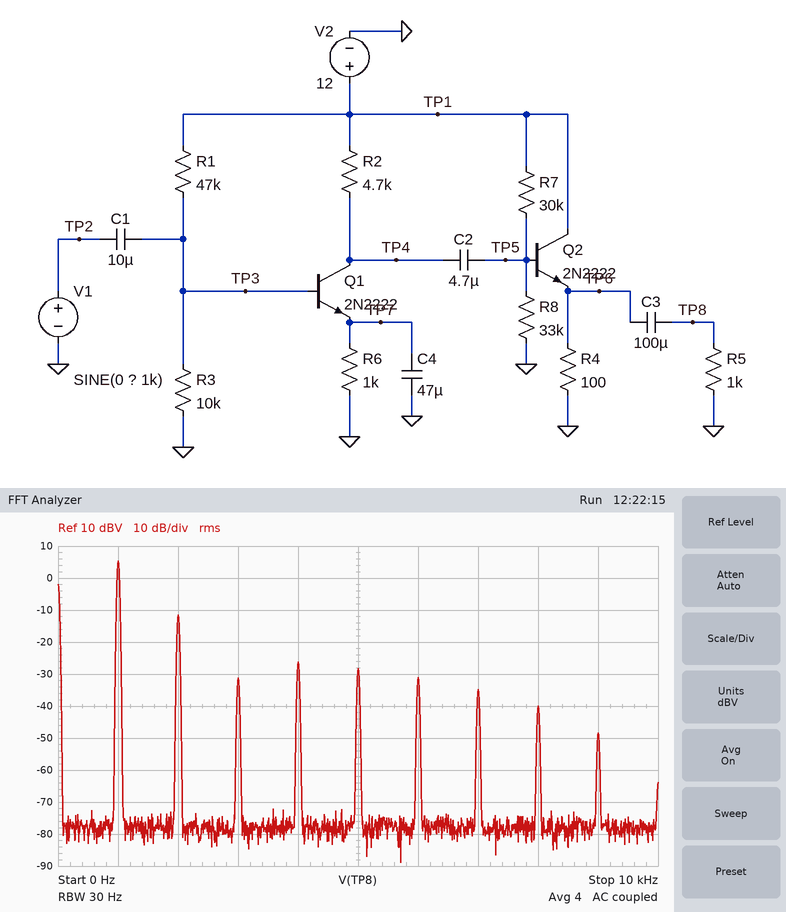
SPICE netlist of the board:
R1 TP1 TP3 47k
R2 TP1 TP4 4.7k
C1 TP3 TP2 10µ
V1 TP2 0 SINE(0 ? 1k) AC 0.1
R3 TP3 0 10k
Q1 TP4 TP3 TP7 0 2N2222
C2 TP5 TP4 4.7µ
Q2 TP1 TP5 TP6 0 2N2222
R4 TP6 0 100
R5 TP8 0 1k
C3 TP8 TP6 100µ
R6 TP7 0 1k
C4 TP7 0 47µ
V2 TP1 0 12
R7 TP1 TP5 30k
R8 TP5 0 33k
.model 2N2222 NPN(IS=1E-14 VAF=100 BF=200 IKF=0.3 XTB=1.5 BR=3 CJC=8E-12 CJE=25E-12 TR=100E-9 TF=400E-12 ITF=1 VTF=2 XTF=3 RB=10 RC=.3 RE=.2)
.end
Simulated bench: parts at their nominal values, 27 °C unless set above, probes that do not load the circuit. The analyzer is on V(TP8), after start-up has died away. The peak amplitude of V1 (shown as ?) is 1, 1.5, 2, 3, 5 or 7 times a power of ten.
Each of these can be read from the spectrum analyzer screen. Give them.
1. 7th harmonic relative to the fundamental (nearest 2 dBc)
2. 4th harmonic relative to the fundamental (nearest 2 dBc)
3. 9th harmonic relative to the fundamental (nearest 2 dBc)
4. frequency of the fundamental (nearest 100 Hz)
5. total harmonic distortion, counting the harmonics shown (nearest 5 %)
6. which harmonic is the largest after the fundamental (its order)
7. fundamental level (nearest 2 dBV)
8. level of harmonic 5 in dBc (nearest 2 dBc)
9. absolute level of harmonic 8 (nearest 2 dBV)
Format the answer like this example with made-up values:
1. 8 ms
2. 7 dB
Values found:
1. -40 dBc
2. -32 dBc
3. -54 dBc
4. 1.0 kHz
5. 15 %
6. 2
7. 6 dBV
8. -34 dBc
9. -40 dBV
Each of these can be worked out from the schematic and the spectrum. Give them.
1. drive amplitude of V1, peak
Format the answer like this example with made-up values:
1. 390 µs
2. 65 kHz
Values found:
1. 20 mV
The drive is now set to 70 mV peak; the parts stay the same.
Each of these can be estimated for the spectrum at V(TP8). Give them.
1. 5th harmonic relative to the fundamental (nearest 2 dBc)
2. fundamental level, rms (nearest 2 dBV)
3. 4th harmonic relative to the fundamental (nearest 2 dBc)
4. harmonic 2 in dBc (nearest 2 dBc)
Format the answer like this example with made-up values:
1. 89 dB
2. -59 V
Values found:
1. -26 dBc
2. 6 dBV
3. -16 dBc
4. -12 dBc
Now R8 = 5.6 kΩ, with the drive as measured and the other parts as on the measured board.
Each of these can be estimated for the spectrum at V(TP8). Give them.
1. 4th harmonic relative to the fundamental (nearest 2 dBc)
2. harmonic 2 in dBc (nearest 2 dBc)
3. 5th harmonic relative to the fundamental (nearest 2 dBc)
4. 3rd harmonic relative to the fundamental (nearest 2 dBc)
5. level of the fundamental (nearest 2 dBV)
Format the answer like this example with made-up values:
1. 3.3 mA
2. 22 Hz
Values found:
1. -28 dBc
2. -26 dBc
3. -36 dBc
4. -18 dBc
5. 0 dBV
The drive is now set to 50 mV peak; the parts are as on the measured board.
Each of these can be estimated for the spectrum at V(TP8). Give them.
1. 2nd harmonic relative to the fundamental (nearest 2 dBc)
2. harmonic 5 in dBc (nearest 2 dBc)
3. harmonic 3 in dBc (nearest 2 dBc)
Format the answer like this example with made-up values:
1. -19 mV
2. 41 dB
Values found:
1. -16 dBc
2. -32 dBc
3. -18 dBc
